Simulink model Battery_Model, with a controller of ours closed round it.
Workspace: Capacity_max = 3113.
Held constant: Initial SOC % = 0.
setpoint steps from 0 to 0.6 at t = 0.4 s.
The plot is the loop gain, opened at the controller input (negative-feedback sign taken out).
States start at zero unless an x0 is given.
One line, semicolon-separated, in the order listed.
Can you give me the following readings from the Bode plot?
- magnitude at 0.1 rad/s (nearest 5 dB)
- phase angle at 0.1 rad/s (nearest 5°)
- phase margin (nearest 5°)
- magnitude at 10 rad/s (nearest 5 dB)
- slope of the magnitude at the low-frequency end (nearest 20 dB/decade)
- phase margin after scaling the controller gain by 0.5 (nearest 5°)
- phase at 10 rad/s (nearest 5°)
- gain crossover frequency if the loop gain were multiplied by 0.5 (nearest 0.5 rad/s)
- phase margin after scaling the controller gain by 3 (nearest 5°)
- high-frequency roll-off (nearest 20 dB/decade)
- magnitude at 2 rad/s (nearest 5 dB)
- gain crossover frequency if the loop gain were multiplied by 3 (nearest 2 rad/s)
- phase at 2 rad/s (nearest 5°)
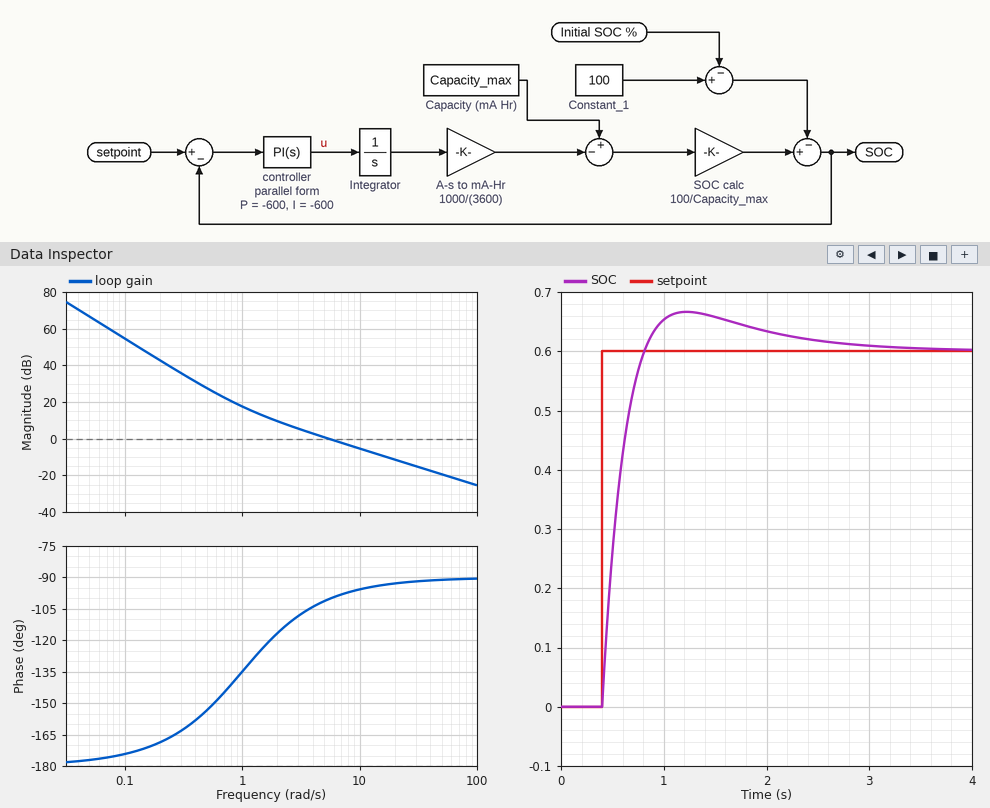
55 dB; -175°; 80°; -5 dB; -40 dB/decade; 70°; -95°; 3.0 rad/s; 85°; -20 dB/decade; 10 dB; 16 rad/s; -115°
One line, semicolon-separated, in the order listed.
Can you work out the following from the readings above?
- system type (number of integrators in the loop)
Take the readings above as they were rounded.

2
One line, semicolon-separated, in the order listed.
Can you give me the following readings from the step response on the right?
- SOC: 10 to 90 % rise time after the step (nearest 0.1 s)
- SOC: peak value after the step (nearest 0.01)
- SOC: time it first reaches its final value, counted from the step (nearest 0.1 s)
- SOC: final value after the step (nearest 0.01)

0.3 s; 0.67; 0.4 s; 0.60
